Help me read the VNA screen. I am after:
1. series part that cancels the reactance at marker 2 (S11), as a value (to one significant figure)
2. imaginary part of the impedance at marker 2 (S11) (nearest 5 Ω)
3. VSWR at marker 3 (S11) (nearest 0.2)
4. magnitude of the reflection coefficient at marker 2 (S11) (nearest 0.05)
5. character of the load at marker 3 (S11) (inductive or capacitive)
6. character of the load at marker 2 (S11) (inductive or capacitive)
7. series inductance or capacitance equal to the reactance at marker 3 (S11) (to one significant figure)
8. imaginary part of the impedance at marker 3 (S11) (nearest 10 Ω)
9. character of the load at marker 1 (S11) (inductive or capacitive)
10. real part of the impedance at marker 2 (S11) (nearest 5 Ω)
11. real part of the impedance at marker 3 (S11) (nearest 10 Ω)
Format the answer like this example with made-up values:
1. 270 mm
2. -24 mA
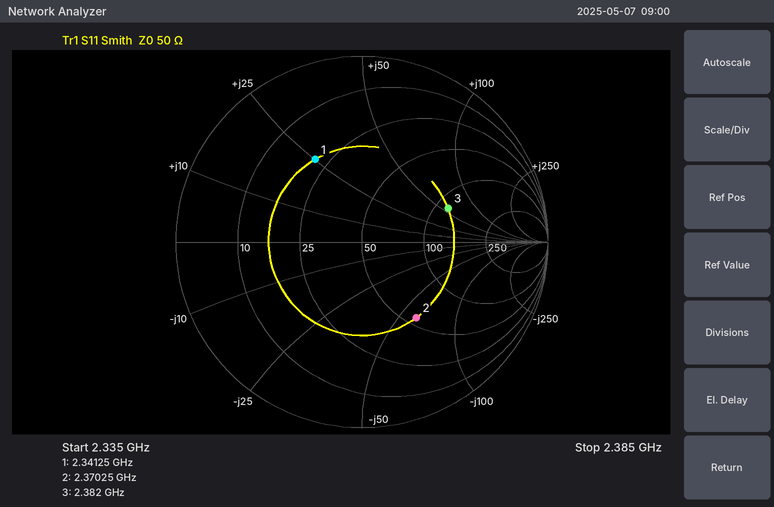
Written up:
1. 4 nH
2. -60 Ω
3. 3.0
4. 0.50
5. inductive
6. capacitive
7. 4 nH
8. +60 Ω
9. inductive
10. 55 Ω
11. 120 Ω
